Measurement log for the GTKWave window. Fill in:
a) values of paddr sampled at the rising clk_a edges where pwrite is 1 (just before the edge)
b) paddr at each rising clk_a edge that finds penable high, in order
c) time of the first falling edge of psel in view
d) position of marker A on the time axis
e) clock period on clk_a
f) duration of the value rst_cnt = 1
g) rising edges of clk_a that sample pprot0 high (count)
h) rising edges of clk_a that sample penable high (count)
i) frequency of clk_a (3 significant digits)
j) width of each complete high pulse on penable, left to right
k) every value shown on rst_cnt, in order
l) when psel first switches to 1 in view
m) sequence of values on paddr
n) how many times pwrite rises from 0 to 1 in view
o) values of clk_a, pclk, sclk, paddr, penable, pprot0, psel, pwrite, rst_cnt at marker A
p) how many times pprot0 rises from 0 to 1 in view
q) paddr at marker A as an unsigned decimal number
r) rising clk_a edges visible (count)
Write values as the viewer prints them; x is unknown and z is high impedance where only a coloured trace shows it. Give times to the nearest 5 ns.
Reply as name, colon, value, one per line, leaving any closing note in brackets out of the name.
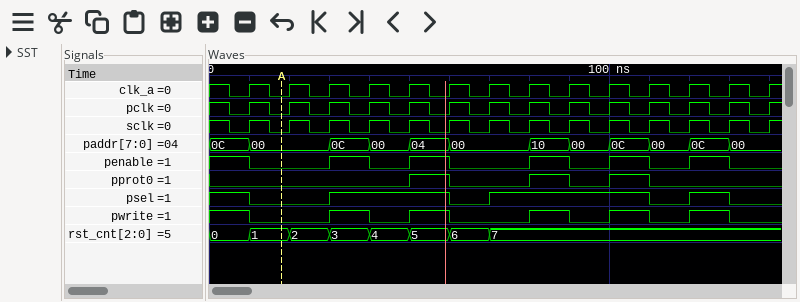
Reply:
values of paddr sampled at the rising clk_a edges where pwrite is 1: 0C, 0C, 04, 10, 0C, 0C
paddr at each rising clk_a edge that finds penable high, in order: 0C, 0C, 04, 10, 0C, 0C
time of the first falling edge of psel in view: 10 ns
position of marker A on the time axis: 20 ns
clock period on clk_a: 10 ns
duration of the value rst_cnt = 1: 10 ns
rising edges of clk_a that sample pprot0 high: 3
rising edges of clk_a that sample penable high: 6
frequency of clk_a: 100 MHz
width of each complete high pulse on penable, left to right: 10 ns, 10 ns, 10 ns, 10 ns, 10 ns
every value shown on rst_cnt, in order: 0, 1, 2, 3, 4, 5, 6, 7
when psel first switches to 1 in view: 30 ns
sequence of values on paddr: 0C, 00, 0C, 00, 04, 00, 10, 00, 0C, 00, 0C, 00
how many times pwrite rises from 0 to 1 in view: 5
values of clk_a, pclk, sclk, paddr, penable, pprot0, psel, pwrite, rst_cnt at marker A: clk_a=0, pclk=0, sclk=0, paddr=00, penable=0, pprot0=0, psel=0, pwrite=0, rst_cnt=1
how many times pprot0 rises from 0 to 1 in view: 3
paddr at marker A as an unsigned decimal number: 0
rising clk_a edges visible: 14
